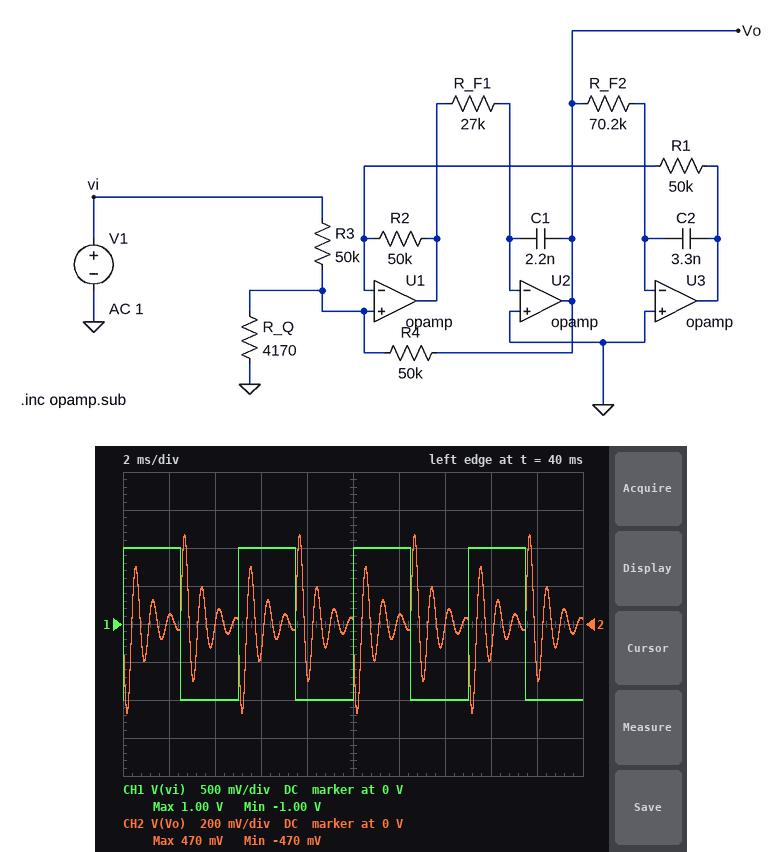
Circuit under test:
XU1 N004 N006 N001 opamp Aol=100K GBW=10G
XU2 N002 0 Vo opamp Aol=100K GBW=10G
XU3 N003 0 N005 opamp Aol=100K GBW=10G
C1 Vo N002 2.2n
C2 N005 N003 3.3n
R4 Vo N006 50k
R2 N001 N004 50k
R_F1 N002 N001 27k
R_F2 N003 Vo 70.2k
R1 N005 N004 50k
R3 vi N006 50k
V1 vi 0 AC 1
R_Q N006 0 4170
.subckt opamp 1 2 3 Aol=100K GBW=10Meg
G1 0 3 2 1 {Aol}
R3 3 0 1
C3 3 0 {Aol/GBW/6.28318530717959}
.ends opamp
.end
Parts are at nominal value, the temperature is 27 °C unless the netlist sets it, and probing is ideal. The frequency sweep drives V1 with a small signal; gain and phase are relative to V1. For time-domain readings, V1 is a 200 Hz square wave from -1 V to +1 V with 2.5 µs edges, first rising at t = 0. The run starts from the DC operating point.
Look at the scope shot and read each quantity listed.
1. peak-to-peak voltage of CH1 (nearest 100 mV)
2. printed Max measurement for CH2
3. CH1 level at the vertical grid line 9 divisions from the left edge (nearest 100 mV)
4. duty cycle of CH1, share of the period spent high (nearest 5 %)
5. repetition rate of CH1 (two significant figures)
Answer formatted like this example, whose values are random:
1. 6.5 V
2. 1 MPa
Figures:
1. 2.0 V
2. 470 mV
3. -1.0 V
4. 50 %
5. 200 Hz
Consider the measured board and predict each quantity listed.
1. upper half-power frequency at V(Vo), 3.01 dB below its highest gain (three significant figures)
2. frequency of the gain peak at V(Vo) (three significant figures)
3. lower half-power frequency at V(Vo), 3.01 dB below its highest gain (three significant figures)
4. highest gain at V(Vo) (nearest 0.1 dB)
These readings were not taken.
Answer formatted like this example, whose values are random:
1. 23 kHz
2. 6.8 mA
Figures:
1. 1.56 kHz
2. 1.36 kHz
3. 1.18 kHz
4. 0 dB
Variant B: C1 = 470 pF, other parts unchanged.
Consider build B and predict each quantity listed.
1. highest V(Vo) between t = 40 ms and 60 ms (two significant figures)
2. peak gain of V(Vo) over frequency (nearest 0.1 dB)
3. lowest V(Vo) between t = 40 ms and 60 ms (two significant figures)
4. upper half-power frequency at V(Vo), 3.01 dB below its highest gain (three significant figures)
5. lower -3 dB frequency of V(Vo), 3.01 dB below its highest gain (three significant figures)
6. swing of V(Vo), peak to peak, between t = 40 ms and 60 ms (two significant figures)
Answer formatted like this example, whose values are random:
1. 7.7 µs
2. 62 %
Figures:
1. 820 mV
2. 0 dB
3. -820 mV
4. 3.97 kHz
5. 2.17 kHz
6. 1.6 V
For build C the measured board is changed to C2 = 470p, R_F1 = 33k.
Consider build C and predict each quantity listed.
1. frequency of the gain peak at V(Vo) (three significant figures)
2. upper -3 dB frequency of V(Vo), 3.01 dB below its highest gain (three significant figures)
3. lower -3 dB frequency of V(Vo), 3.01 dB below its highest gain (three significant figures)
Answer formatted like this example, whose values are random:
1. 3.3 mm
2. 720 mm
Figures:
1. 3.25 kHz
2. 3.41 kHz
3. 3.10 kHz
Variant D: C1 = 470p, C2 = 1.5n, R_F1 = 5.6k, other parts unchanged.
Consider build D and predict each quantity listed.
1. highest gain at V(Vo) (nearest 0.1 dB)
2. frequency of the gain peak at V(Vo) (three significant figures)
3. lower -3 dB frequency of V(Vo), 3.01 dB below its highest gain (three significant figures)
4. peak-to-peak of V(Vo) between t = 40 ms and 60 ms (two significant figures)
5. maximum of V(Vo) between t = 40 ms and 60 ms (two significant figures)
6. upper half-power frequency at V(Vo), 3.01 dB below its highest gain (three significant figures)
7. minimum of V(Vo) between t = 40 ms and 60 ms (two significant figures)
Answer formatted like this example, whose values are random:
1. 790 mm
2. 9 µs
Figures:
1. 0 dB
2. 9.56 kHz
3. 6.17 kHz
4. 2.1 V
5. 1.0 V
6. 14.8 kHz
7. -1.0 V
